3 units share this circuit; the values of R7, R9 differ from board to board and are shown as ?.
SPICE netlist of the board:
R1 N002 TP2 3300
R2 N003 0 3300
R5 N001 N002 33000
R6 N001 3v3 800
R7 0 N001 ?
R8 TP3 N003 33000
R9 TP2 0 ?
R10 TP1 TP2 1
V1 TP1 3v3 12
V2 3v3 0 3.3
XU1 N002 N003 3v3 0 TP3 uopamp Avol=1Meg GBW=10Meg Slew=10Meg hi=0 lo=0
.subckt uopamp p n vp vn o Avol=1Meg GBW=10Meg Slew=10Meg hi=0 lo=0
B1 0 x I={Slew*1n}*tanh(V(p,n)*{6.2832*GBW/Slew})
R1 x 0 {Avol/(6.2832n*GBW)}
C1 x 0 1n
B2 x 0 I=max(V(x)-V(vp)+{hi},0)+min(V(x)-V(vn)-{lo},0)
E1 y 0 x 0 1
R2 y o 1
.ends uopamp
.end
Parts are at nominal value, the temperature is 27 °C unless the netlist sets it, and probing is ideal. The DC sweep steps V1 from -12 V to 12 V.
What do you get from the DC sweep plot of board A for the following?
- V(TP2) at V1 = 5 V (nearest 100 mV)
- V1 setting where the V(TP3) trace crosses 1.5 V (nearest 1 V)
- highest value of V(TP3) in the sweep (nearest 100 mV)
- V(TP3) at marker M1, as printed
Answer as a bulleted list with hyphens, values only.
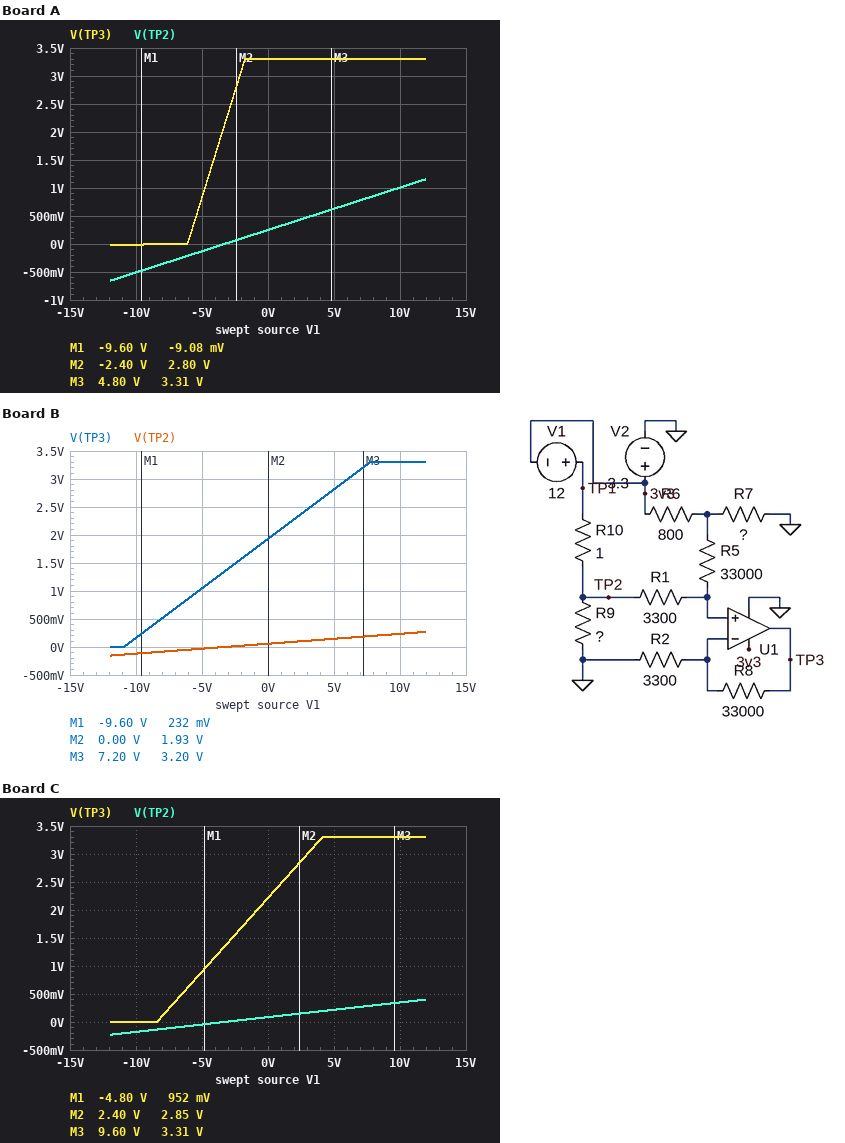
- 600 mV
- -4 V
- 3.3 V
- -9.08 mV
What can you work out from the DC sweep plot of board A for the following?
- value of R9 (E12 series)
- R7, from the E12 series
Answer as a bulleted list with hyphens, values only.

- 0.082 Ω
- 1.5 kΩ
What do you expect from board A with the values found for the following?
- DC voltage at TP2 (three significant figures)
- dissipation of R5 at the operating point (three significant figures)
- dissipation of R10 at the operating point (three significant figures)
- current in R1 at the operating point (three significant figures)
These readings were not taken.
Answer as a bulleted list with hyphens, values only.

- 1.16 V
- 24.0 µW
- 200 W
- 27.0 µA
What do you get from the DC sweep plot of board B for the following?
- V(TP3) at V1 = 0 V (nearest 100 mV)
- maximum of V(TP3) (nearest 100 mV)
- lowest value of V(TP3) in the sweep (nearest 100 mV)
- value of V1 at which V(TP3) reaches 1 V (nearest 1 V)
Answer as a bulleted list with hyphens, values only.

- 1.9 V
- 3.3 V
- 0 V
- -5 V
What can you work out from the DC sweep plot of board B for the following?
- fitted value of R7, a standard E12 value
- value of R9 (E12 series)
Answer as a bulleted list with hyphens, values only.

- 560 Ω
- 0.018 Ω
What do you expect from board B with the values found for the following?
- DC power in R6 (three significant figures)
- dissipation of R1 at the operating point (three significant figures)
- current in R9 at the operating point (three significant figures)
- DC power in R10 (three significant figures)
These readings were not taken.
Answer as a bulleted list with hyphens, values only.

- 4.76 mW
- 2.91 µW
- 15.0 A
- 226 W
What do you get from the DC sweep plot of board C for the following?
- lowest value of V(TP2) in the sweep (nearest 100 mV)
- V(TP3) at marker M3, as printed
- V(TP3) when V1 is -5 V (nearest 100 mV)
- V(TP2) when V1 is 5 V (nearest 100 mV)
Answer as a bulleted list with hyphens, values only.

- -200 mV
- 3.31 V
- 900 mV
- 200 mV
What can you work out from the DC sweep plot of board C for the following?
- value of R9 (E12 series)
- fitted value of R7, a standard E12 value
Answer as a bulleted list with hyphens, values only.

- 0.027 Ω
- 560 Ω
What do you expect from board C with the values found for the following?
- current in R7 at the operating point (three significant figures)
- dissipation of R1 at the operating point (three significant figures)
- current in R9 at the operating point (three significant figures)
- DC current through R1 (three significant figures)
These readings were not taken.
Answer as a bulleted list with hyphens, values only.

- 2.41 mA
- 2.25 µW
- 14.9 A
- 26.1 µA
